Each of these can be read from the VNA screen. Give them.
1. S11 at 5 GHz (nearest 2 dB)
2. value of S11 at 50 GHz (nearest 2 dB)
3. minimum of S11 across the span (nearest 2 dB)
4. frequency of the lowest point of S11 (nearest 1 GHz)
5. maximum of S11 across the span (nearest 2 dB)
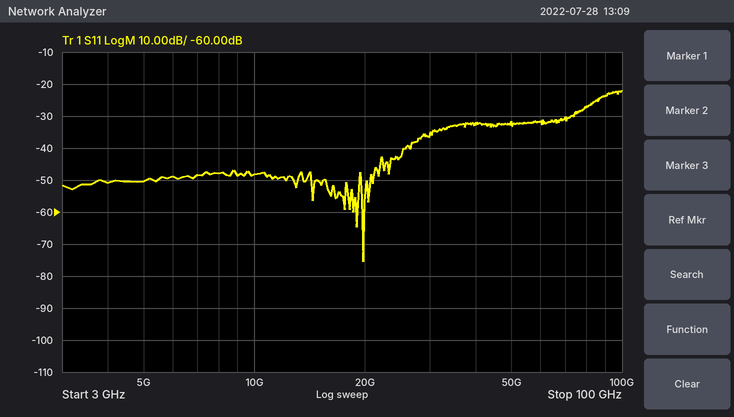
-50 dB
-32 dB
-76 dB
20 GHz
-22 dB
